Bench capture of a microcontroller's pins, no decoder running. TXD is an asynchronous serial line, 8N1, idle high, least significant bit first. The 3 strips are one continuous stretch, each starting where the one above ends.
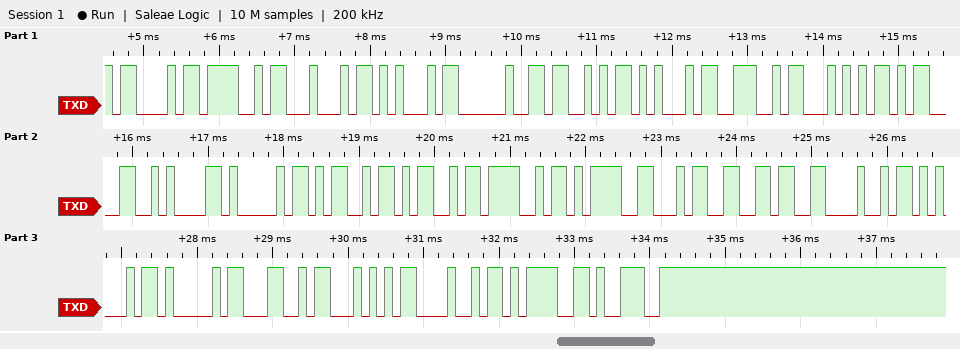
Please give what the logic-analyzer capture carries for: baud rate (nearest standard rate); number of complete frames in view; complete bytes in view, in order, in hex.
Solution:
9600 baud
26
43 4F 44 45 20 53 45 4E 54 0D 0A 41 4D 4D 4F 3D 34 36 48 45 41 4C 54 48 3D 39
